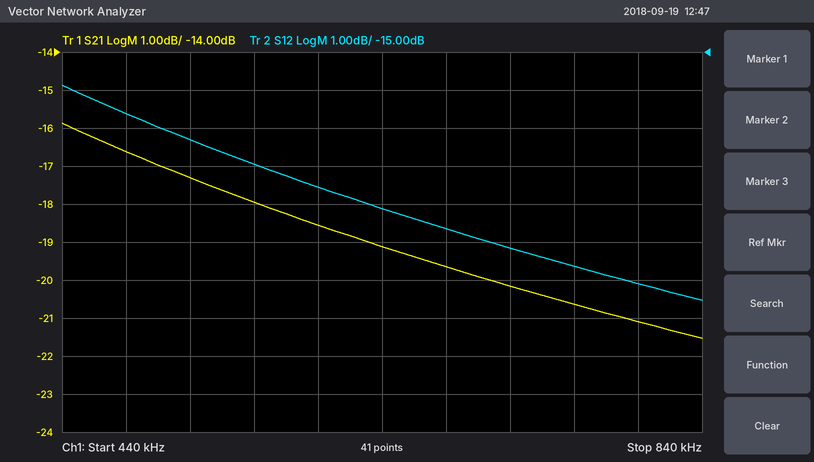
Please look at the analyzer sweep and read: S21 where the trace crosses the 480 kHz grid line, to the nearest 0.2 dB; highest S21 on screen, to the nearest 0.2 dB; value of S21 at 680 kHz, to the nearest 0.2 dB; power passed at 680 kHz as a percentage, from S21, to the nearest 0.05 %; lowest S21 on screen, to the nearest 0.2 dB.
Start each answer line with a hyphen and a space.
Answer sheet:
- -16.6 dB
- -15.8 dB
- -19.6 dB
- 1.10 %
- -21.6 dB
